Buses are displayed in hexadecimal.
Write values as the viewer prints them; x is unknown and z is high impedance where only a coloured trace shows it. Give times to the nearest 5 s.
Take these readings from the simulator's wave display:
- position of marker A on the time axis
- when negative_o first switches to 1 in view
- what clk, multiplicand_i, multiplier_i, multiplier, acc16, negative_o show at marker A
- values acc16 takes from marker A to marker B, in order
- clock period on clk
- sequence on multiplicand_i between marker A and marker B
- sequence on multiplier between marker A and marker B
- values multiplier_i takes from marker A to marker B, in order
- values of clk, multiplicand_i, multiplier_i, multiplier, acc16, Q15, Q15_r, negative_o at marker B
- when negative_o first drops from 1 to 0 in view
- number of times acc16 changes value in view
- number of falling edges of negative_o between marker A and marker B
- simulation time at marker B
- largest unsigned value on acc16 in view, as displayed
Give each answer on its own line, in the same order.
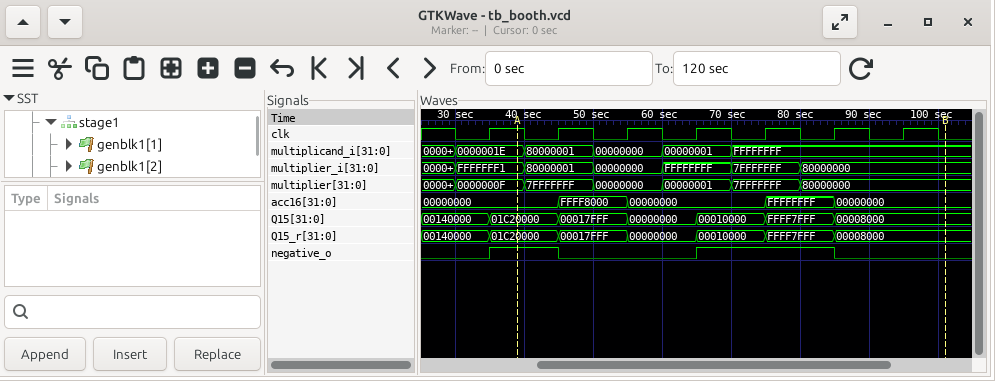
40 s
35 s
clk=1, multiplicand_i=0000001E, multiplier_i=FFFFFFF1, multiplier=0000000F, acc16=00000000, negative_o=1
00000000, FFFF8000, 00000000, FFFFFFFF, 00000000
10 s
0000001E, 80000001, 00000000, 00000001, FFFFFFFF
0000000F, 7FFFFFFF, 00000000, 00000001, 7FFFFFFF, 80000000
FFFFFFF1, 80000001, 00000000, FFFFFFFF, 7FFFFFFF, 80000000
clk=0, multiplicand_i=FFFFFFFF, multiplier_i=80000000, multiplier=80000000, acc16=00000000, Q15=00008000, Q15_r=00008000, negative_o=0
45 s
4
2
100 s
FFFFFFFF
